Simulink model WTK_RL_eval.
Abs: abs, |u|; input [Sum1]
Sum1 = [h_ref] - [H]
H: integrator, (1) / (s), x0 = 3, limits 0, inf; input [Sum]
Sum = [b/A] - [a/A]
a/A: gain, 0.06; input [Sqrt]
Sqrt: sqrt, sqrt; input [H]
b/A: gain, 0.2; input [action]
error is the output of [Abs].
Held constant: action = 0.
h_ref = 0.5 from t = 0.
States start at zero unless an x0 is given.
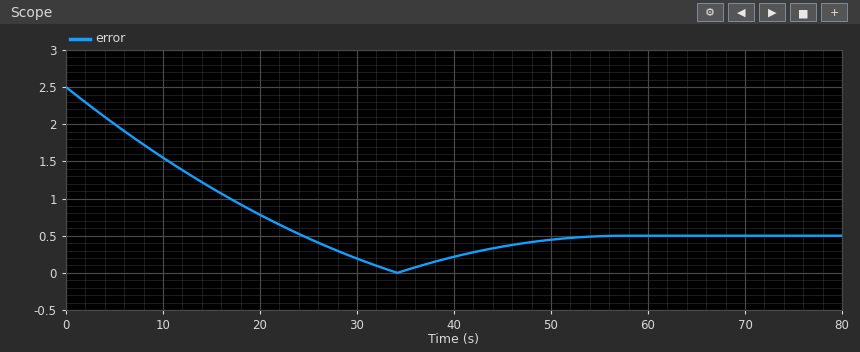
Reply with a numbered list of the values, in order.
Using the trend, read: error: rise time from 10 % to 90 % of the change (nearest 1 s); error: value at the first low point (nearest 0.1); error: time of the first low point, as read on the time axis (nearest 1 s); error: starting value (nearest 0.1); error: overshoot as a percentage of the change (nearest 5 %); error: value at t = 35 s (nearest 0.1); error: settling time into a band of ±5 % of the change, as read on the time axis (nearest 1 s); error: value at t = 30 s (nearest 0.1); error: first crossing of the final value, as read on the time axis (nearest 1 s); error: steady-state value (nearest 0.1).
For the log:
1. 19 s
2. 0.0
3. 34 s
4. 2.5
5. 25 %
6. 0.0
7. 47 s
8. 0.2
9. 24 s
10. 0.5
